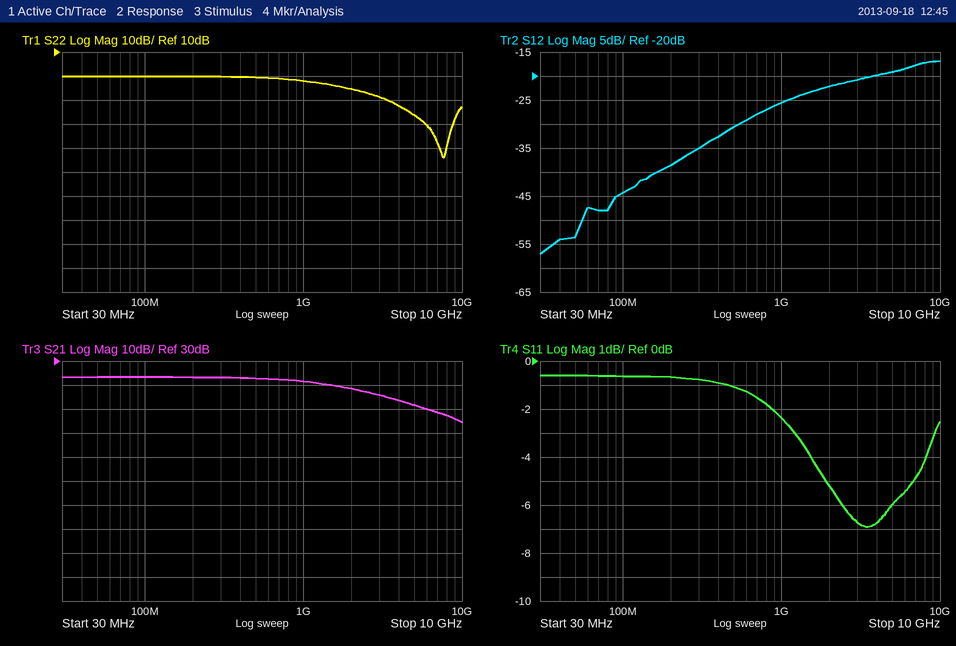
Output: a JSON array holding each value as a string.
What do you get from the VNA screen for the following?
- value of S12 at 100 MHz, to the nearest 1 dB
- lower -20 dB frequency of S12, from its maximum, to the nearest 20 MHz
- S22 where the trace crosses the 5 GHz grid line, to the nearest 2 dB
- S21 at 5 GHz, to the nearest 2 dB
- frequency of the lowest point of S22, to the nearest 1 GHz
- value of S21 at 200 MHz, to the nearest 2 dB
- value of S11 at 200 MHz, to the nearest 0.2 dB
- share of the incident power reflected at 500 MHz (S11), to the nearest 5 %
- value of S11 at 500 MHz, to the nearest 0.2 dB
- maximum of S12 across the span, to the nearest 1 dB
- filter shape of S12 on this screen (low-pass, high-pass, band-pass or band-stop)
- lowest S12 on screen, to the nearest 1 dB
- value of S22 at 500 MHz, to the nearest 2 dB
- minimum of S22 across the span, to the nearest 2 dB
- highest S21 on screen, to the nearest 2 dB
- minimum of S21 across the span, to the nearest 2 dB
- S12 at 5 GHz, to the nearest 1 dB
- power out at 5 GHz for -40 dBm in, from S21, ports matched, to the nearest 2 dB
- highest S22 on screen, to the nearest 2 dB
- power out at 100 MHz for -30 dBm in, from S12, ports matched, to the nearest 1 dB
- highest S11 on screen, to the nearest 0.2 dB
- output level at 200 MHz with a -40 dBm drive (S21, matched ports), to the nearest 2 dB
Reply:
["-44 dB", "240 MHz", "-16 dB", "12 dB", "8 GHz", "24 dB", "-0.6 dB", "80 %", "-1.0 dB", "-17 dB", "high-pass", "-57 dB", "0 dB", "-34 dB", "24 dB", "4 dB", "-19 dB", "-28 dBm", "0 dB", "-74 dBm", "-0.6 dB", "-16 dBm"]
